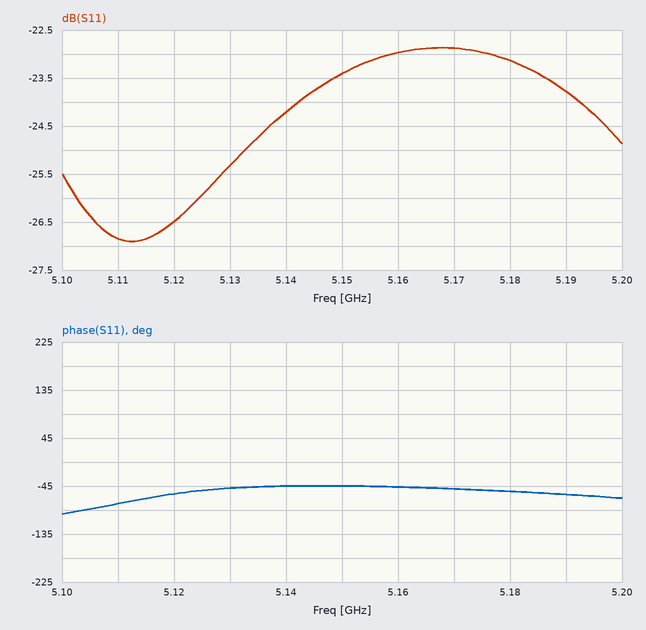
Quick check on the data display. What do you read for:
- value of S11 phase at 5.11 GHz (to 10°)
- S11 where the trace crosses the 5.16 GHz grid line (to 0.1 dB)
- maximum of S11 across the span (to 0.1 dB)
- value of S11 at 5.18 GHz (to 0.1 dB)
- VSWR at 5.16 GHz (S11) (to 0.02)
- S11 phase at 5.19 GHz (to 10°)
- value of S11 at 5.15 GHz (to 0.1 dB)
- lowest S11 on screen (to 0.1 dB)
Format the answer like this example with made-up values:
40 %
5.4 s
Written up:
-80°
-23.0 dB
-22.9 dB
-23.1 dB
1.16
-60°
-23.4 dB
-26.9 dB
